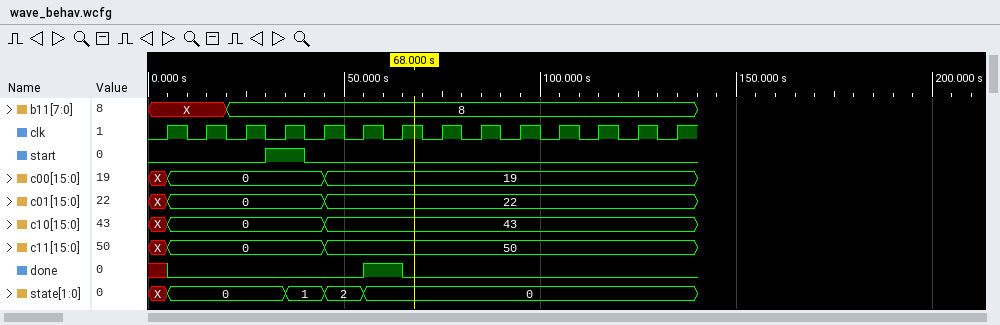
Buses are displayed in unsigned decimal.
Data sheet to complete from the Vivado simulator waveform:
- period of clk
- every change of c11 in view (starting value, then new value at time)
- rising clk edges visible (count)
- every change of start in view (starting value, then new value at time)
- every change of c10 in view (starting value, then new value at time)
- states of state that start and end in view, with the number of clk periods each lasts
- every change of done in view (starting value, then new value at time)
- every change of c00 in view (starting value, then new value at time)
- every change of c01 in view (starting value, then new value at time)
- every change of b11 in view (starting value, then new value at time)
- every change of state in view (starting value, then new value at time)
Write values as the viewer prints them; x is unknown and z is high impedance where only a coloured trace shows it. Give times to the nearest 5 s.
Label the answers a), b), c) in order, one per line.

a) 10 s
b) X, 0 at 5 s, 50 at 45 s
c) 14
d) 0, 1 at 30 s, 0 at 40 s
e) X, 0 at 5 s, 43 at 45 s
f) 0: 3, 1: 1, 2: 1
g) x, 0 at 5 s, 1 at 55 s, 0 at 65 s
h) X, 0 at 5 s, 19 at 45 s
i) X, 0 at 5 s, 22 at 45 s
j) X, 8 at 20 s
k) X, 0 at 5 s, 1 at 35 s, 2 at 45 s, 0 at 55 s
